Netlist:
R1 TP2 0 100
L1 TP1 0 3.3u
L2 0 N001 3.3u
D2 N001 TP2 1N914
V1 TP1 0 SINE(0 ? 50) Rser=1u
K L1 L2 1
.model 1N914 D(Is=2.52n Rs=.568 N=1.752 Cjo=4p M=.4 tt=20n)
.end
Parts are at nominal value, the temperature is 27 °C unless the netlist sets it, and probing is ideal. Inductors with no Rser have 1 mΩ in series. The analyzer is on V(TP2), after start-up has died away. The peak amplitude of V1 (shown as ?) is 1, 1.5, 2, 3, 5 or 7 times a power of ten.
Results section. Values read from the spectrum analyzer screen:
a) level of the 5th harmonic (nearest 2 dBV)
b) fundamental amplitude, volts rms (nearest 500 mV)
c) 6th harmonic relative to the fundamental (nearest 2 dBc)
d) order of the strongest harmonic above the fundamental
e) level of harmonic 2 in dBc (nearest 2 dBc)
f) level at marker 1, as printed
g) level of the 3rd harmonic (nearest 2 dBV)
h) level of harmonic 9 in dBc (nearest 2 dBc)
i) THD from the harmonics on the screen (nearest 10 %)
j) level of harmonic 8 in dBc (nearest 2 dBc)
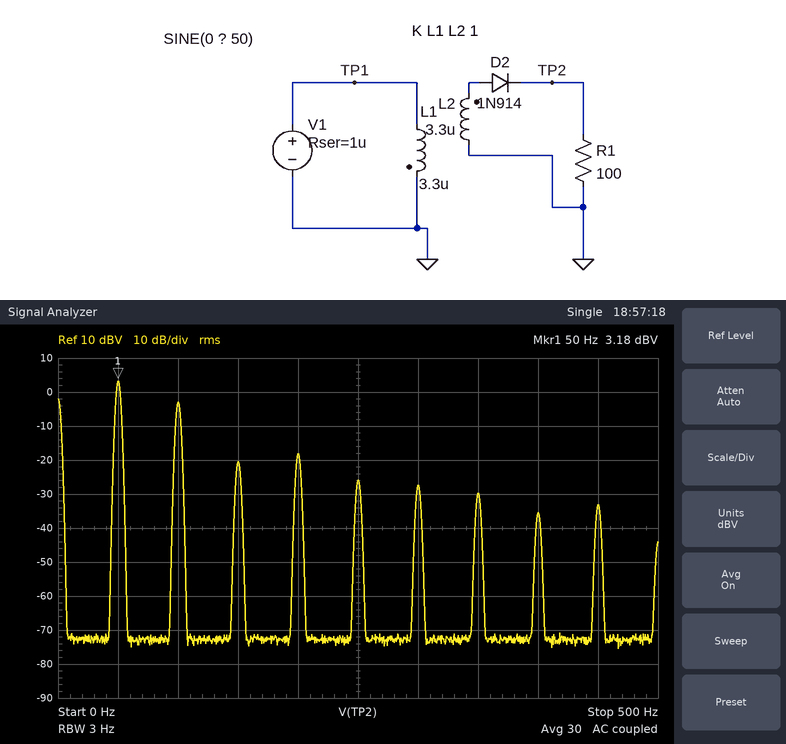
-26 dBV
1.5 V
-30 dBc
2
-6 dBc
3.18 dBV
-20 dBV
-36 dBc
50 %
-38 dBc
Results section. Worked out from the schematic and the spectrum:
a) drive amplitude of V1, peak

7 V
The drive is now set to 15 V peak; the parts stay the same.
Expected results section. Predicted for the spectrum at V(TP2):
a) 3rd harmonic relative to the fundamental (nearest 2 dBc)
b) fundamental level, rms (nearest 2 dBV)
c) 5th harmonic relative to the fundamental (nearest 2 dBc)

-30 dBc
10 dBV
-36 dBc
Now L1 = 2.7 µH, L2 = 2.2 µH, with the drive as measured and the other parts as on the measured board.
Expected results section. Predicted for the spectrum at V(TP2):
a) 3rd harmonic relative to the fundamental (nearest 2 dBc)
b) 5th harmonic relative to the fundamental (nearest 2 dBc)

-22 dBc
-28 dBc
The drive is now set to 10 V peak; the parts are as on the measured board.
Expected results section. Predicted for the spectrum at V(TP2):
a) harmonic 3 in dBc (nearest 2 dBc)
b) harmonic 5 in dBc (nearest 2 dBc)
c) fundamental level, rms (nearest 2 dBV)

-26 dBc
-32 dBc
6 dBV
